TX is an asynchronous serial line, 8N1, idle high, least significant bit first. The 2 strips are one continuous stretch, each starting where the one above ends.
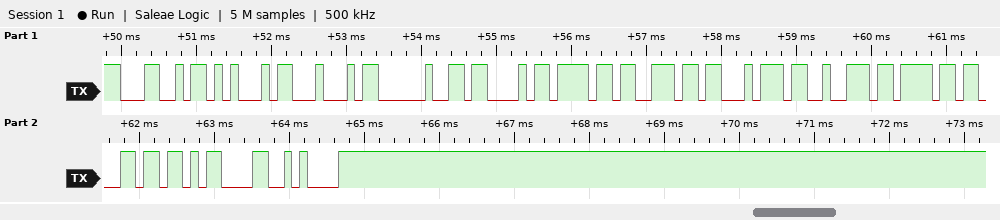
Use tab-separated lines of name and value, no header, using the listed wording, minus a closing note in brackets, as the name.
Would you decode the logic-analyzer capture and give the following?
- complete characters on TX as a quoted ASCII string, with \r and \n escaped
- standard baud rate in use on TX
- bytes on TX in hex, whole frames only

complete characters on TX as a quoted ASCII string, with \r and \n escaped	"LED Control\r\n"
standard baud rate in use on TX	9600 baud
bytes on TX in hex, whole frames only	0x4C 0x45 0x44 0x20 0x43 0x6F 0x6E 0x74 0x72 0x6F 0x6C 0x0D 0x0A
